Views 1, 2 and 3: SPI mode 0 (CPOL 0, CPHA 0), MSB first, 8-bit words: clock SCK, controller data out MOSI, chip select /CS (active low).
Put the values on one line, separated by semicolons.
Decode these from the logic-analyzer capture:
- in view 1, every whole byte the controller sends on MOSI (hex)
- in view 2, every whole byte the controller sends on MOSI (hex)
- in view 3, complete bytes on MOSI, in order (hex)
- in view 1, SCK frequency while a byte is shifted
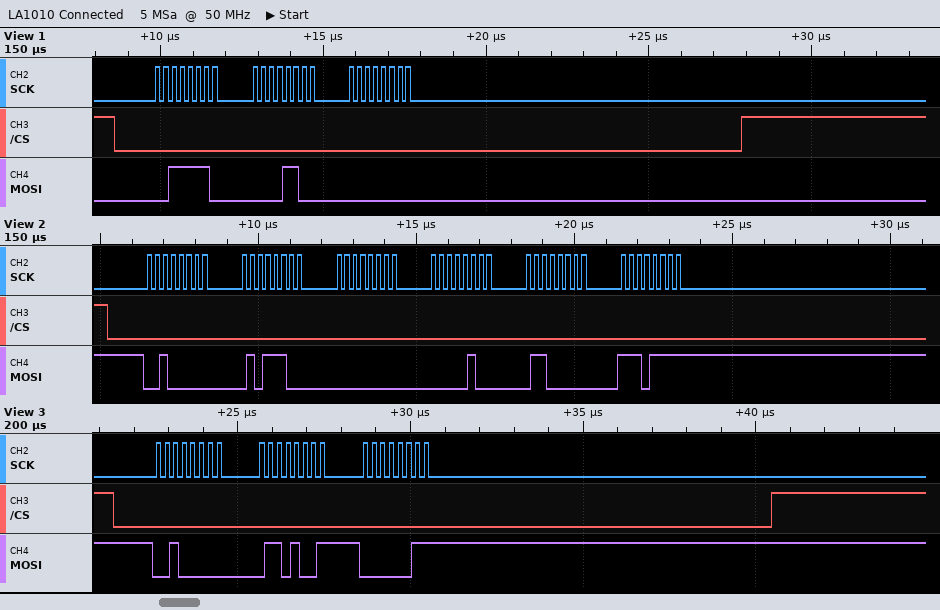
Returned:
0x3E 0x0C 0x00; 0x20 0x5C 0x00 0x04 0x60 0xEF; 20 69 03; 4 MHz
